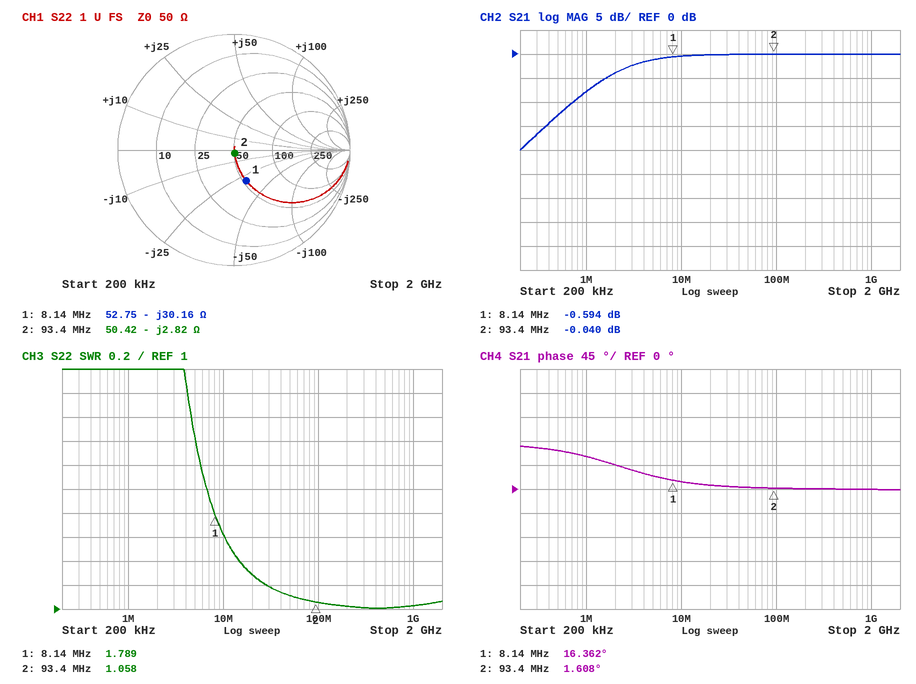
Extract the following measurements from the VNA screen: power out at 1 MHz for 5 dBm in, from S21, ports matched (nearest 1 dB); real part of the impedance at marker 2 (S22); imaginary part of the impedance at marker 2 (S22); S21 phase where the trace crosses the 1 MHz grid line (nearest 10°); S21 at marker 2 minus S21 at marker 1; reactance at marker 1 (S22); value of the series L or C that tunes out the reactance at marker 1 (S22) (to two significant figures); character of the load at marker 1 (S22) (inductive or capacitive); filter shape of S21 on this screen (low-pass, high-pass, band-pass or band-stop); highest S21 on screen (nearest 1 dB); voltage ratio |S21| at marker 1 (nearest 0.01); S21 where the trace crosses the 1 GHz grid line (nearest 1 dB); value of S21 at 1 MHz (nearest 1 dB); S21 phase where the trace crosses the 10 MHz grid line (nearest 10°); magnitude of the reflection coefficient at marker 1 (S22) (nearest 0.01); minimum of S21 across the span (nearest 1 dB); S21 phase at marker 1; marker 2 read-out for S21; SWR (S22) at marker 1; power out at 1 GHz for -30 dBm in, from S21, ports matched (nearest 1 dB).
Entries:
-3 dBm
50.42 Ω
-2.82 Ω
60°
0.554 dB
-30.16 Ω
590 nH
capacitive
high-pass
0 dB
0.93
0 dB
-8 dB
10°
0.28
-20 dB
16.362°
-0.040 dB
1.789
-30 dBm
